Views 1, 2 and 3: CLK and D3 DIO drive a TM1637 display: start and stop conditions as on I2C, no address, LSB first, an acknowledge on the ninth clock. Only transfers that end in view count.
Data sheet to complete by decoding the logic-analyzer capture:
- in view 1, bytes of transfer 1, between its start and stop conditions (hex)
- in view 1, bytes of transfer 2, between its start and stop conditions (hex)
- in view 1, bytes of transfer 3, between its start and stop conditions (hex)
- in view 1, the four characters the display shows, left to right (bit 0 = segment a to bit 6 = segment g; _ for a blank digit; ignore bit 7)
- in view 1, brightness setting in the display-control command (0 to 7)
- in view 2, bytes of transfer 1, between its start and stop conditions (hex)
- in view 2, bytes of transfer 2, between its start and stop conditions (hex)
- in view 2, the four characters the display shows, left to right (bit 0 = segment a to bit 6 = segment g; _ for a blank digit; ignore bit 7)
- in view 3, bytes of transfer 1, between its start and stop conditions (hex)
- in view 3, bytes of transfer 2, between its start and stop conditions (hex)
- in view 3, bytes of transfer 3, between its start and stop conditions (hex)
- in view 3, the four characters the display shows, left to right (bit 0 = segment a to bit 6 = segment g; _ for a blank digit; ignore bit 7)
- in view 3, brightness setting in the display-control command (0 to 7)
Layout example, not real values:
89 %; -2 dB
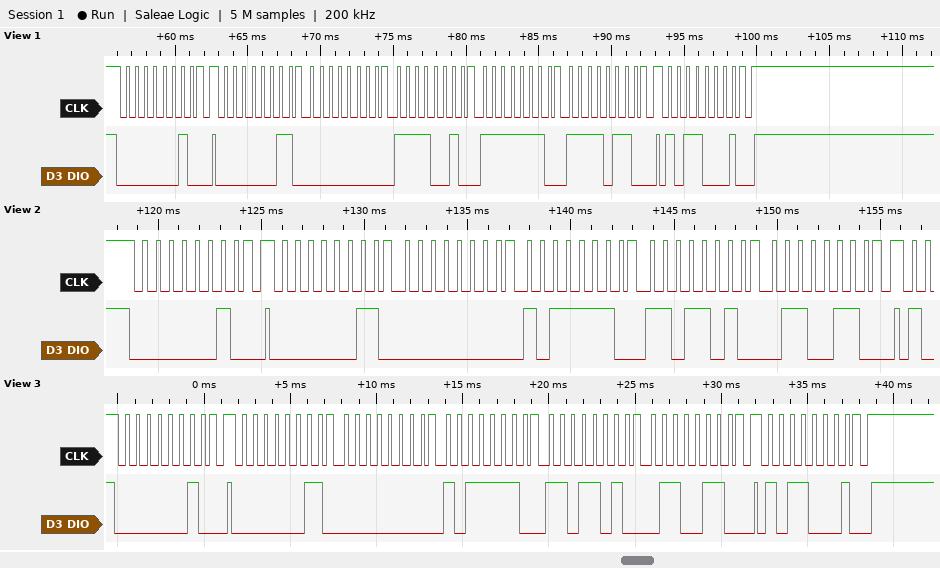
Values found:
40; C0 00 4F 7F 6F; 8D; _389; 5; 40; C0 00 7D 5B 66; _624; 40; C0 00 7D 5B 66; 8D; _624; 5
